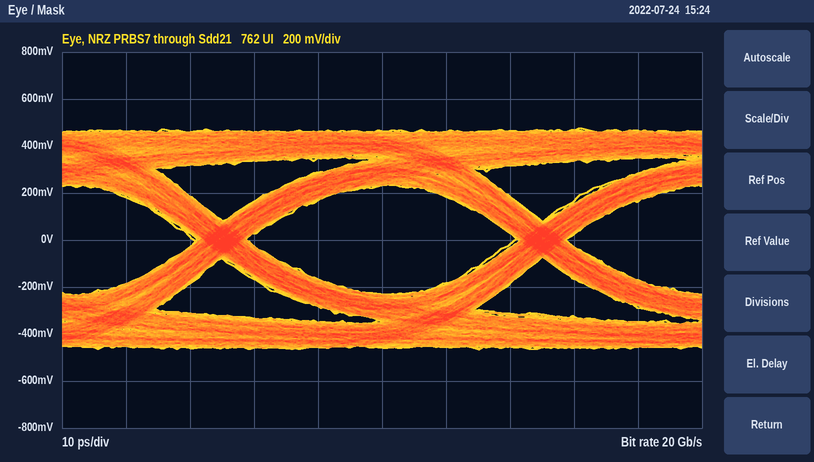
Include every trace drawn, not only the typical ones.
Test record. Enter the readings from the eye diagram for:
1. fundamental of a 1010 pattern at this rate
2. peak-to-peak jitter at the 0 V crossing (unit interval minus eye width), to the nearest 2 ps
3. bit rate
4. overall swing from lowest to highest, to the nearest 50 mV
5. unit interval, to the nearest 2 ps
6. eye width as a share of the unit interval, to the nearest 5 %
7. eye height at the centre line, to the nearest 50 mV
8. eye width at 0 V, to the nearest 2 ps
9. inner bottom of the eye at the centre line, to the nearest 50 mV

10 GHz
8 ps
20 Gb/s
950 mV
50 ps
85 %
450 mV
42 ps
-250 mV
